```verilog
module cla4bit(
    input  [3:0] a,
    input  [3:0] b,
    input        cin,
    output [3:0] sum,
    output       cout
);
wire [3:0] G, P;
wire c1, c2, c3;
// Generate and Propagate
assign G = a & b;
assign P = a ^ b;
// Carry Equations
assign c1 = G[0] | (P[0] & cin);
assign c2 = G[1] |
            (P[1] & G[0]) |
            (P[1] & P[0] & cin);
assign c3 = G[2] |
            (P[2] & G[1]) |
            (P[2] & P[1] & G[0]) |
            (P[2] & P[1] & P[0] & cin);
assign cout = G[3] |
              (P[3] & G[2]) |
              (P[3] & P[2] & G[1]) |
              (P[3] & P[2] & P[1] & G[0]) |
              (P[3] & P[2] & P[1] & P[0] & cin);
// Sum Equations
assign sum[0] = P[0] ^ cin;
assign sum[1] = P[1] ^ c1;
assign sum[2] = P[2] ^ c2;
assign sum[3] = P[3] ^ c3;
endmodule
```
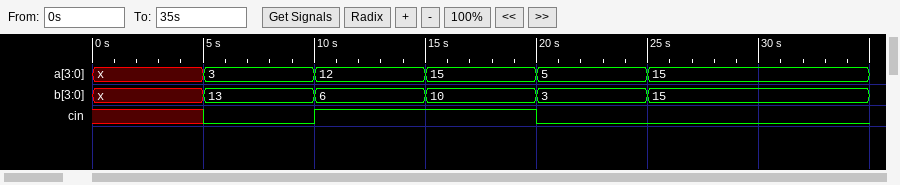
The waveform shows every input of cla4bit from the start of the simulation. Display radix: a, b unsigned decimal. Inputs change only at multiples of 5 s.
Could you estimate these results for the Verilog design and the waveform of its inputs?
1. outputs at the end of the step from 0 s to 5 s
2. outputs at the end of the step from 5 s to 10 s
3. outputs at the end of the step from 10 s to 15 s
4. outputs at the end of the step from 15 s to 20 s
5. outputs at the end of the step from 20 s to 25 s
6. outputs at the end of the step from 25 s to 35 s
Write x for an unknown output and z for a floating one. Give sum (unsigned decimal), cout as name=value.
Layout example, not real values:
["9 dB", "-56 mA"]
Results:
["sum=x, cout=x", "sum=0, cout=1", "sum=3, cout=1", "sum=10, cout=1", "sum=8, cout=0", "sum=14, cout=1"]
